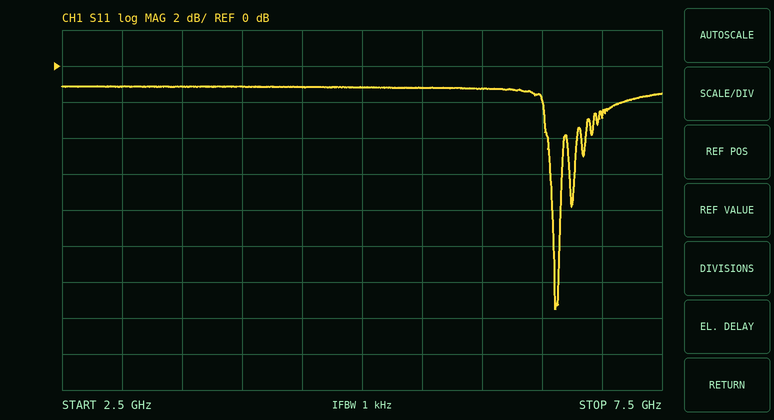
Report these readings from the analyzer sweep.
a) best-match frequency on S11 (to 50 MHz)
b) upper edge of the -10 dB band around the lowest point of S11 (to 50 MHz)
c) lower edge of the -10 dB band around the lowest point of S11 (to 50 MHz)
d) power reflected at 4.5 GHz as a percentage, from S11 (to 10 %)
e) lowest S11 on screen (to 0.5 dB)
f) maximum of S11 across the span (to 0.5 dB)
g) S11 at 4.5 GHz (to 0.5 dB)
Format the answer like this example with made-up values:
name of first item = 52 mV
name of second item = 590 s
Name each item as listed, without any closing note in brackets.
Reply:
best-match frequency on S11 = 6.60 GHz
upper edge of the -10 dB band around the lowest point of S11 = 6.65 GHz
lower edge of the -10 dB band around the lowest point of S11 = 6.60 GHz
power reflected at 4.5 GHz as a percentage, from S11 = 80 %
lowest S11 on screen = -13.5 dB
maximum of S11 across the span = -1.0 dB
S11 at 4.5 GHz = -1.0 dB
